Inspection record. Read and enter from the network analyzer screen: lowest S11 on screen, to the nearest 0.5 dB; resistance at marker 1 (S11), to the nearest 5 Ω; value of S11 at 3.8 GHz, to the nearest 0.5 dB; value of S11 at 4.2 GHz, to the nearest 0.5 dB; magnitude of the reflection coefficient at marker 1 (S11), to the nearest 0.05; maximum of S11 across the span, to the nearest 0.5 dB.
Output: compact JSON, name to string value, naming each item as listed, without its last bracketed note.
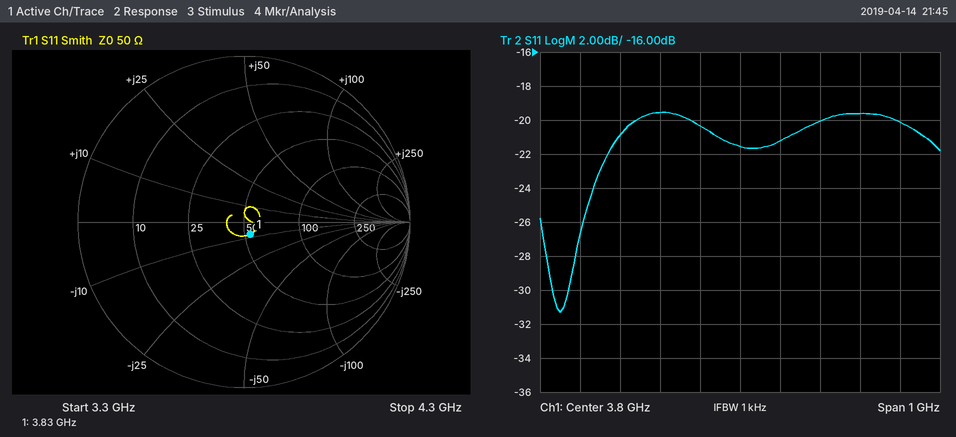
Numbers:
{"lowest S11 on screen, to the nearest 0.5 dB": "-31.5 dB", "resistance at marker 1 (S11), to the nearest 5 Ω": "55 Ω", "value of S11 at 3.8 GHz, to the nearest 0.5 dB": "-21.5 dB", "value of S11 at 4.2 GHz, to the nearest 0.5 dB": "-20.0 dB", "magnitude of the reflection coefficient at marker 1 (S11), to the nearest 0.05": "0.10", "maximum of S11 across the span, to the nearest 0.5 dB": "-19.5 dB"}
